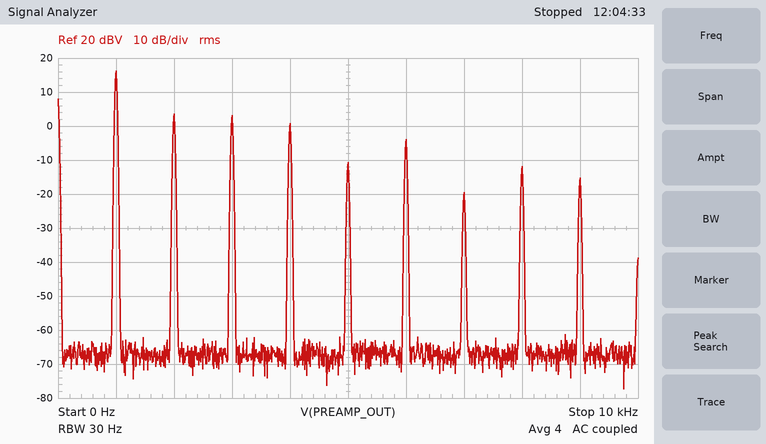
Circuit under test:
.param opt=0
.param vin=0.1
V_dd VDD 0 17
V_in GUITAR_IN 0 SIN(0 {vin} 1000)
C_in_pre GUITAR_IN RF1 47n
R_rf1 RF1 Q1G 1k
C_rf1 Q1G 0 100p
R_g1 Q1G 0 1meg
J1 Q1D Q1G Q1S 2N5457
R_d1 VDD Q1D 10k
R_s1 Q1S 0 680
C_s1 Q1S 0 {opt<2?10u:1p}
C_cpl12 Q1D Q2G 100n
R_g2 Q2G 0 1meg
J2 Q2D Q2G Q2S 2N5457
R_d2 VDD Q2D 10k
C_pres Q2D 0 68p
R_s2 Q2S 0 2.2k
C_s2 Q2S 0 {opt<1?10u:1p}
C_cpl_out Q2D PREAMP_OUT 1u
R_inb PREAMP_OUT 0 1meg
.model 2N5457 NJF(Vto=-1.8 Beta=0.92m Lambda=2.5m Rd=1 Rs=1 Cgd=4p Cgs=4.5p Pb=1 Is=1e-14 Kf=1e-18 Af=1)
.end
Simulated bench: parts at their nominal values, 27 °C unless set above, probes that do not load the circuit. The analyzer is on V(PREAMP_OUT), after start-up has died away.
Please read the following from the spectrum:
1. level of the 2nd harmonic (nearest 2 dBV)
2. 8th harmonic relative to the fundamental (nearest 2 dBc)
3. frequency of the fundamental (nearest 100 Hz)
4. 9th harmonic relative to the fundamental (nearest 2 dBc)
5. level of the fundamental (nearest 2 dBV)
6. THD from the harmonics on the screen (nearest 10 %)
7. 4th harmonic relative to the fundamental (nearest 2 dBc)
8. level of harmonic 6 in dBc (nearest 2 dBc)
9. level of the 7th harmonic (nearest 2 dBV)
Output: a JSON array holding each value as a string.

["4 dBV", "-28 dBc", "1.0 kHz", "-32 dBc", "16 dBV", "40 %", "-16 dBc", "-20 dBc", "-20 dBV"]
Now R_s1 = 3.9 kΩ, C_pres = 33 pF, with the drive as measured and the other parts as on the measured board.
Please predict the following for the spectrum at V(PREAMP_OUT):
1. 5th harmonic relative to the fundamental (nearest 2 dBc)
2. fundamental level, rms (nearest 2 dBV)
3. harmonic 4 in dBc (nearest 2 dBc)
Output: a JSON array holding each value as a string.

["-34 dBc", "16 dBV", "-20 dBc"]
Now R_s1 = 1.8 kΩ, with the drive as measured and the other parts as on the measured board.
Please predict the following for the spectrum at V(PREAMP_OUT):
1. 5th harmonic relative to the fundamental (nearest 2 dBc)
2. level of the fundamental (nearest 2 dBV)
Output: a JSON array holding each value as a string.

["-44 dBc", "16 dBV"]
